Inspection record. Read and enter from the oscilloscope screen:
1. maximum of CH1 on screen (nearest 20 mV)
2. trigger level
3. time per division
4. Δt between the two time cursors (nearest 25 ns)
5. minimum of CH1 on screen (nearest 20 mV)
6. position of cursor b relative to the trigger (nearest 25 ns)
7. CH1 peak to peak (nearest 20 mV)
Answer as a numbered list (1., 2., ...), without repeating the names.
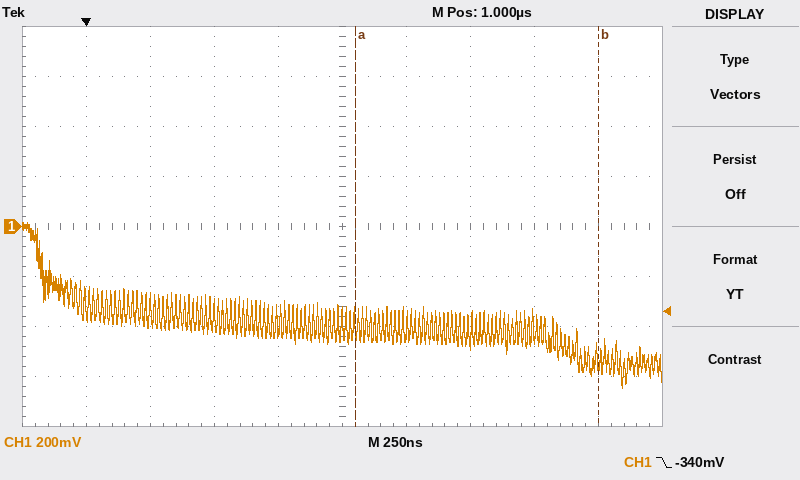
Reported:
1. 20 mV
2. -340 mV
3. 250 ns
4. 950 ns
5. -640 mV
6. +2.000 µs
7. 660 mV
